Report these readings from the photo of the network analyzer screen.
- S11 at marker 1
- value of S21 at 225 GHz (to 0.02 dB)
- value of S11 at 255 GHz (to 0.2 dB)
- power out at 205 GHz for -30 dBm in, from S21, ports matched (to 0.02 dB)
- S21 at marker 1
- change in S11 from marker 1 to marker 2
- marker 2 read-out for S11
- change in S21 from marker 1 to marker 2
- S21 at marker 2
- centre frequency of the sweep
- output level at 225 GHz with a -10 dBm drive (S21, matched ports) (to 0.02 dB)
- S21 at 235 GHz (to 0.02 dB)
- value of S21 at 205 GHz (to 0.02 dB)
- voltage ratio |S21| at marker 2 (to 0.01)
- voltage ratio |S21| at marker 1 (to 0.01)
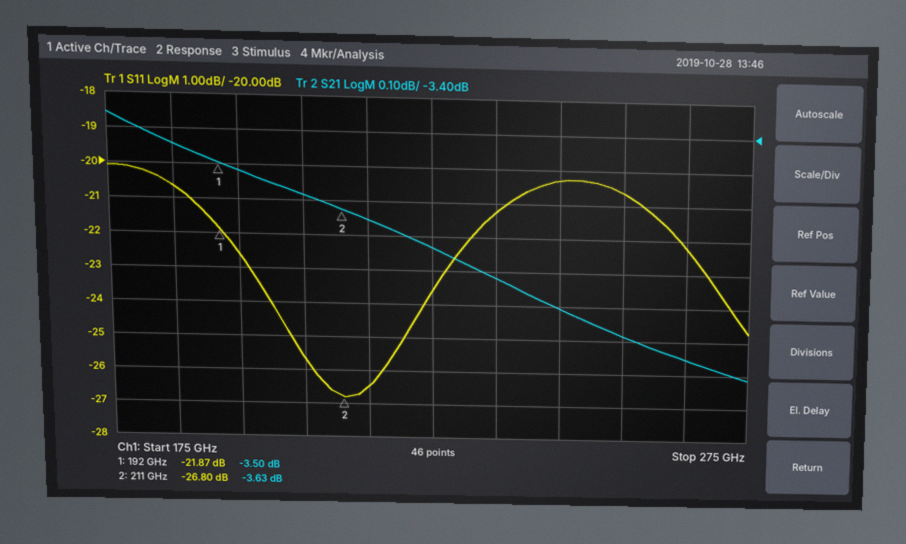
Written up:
-21.87 dB
-3.74 dB
-20.6 dB
-33.58 dBm
-3.50 dB
-4.93 dB
-26.80 dB
-0.13 dB
-3.63 dB
225 GHz
-13.74 dBm
-3.82 dB
-3.58 dB
0.66
0.67
